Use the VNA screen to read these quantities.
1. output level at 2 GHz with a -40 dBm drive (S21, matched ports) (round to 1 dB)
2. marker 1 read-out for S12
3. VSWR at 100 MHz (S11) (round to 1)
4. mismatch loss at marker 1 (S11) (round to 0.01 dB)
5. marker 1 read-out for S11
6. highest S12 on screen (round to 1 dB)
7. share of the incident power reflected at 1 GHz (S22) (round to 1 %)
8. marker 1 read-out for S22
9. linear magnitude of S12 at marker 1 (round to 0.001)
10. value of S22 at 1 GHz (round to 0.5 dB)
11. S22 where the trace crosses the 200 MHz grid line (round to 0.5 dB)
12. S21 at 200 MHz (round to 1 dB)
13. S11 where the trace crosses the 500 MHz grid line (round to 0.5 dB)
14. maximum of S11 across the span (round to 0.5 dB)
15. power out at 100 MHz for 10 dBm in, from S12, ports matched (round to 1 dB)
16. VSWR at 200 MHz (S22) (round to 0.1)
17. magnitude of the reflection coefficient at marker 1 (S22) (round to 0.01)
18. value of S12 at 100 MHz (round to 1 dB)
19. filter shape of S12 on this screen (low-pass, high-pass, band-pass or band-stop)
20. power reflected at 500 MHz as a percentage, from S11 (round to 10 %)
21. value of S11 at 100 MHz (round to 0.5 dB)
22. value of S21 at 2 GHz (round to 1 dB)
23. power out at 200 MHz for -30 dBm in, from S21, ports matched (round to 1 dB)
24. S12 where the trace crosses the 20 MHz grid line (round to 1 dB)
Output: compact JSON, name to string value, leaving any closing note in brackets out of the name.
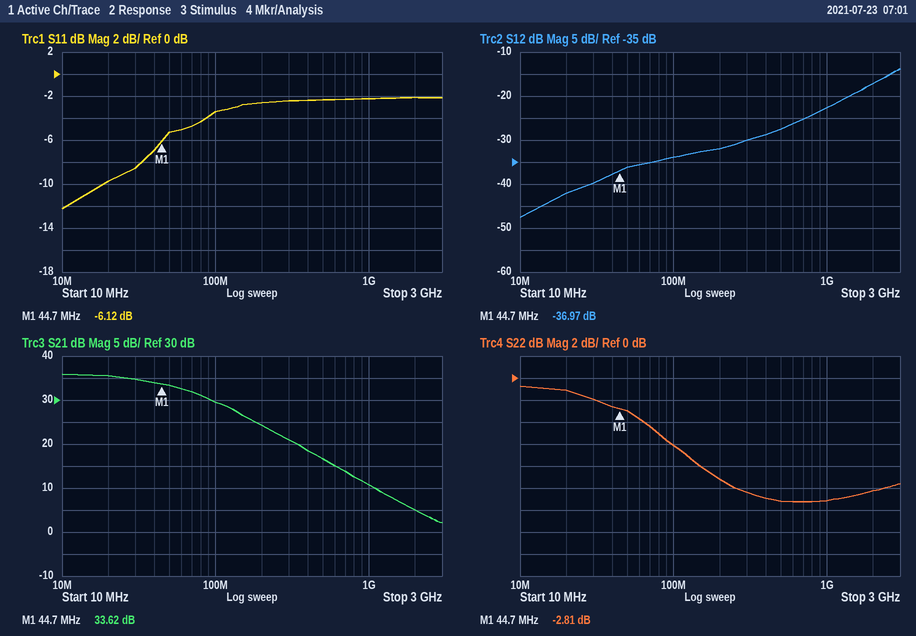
{"output level at 2 GHz with a -40 dBm drive (S21, matched ports)": "-35 dBm", "marker 1 read-out for S12": "-36.97 dB", "VSWR at 100 MHz (S11)": "5", "mismatch loss at marker 1 (S11)": "1.22 dB", "marker 1 read-out for S11": "-6.12 dB", "highest S12 on screen": "-14 dB", "share of the incident power reflected at 1 GHz (S22)": "8 %", "marker 1 read-out for S22": "-2.81 dB", "linear magnitude of S12 at marker 1": "0.014", "value of S22 at 1 GHz": "-11.0 dB", "S22 where the trace crosses the 200 MHz grid line": "-9.0 dB", "S21 at 200 MHz": "24 dB", "S11 where the trace crosses the 500 MHz grid line": "-2.5 dB", "maximum of S11 across the span": "-2.0 dB", "power out at 100 MHz for 10 dBm in, from S12, ports matched": "-24 dBm", "VSWR at 200 MHz (S22)": "2.1", "magnitude of the reflection coefficient at marker 1 (S22)": "0.72", "value of S12 at 100 MHz": "-34 dB", "filter shape of S12 on this screen": "high-pass", "power reflected at 500 MHz as a percentage, from S11": "60 %", "value of S11 at 100 MHz": "-3.5 dB", "value of S21 at 2 GHz": "5 dB", "power out at 200 MHz for -30 dBm in, from S21, ports matched": "-6 dBm", "S12 where the trace crosses the 20 MHz grid line": "-42 dB"}
